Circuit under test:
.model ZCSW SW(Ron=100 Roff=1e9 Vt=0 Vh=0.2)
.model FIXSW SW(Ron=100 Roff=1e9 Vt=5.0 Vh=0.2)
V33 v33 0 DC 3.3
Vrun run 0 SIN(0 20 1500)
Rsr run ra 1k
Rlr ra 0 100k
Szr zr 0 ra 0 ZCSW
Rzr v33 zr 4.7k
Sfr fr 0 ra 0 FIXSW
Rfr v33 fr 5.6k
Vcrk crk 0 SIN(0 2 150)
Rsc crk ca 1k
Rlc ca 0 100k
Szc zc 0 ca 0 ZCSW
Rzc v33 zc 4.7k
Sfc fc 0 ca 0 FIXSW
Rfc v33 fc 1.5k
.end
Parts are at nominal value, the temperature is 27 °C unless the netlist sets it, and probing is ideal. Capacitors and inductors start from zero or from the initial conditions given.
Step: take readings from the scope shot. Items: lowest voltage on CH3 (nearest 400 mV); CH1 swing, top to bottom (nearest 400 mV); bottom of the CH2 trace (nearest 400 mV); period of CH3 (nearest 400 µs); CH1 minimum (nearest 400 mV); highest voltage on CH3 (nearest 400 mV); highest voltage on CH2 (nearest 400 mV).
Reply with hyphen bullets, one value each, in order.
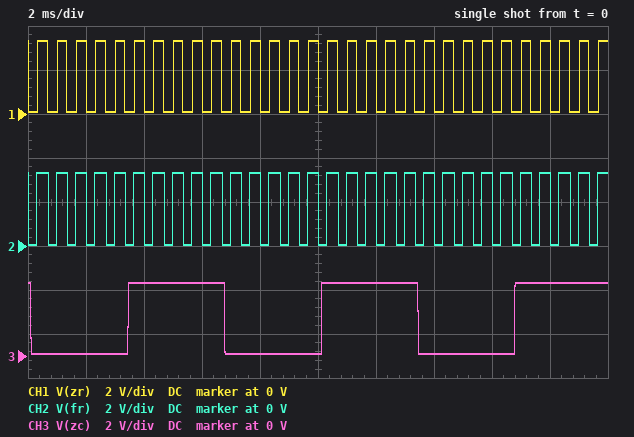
- 0 V
- 3.2 V
- 0 V
- 6.8 ms
- 0 V
- 3.2 V
- 3.2 V
